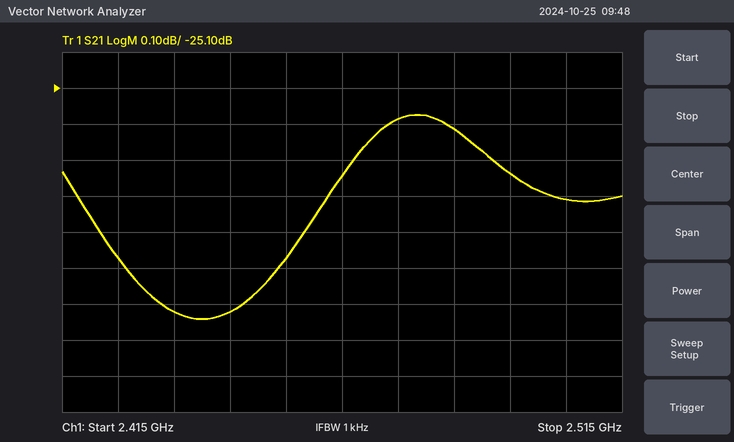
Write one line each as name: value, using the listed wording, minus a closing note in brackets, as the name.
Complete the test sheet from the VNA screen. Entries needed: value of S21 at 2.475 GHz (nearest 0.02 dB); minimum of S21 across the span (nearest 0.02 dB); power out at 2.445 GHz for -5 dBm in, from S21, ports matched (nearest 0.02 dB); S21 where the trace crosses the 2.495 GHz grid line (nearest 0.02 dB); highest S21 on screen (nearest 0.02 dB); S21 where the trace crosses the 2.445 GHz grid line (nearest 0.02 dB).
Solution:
value of S21 at 2.475 GHz: -25.18 dB
minimum of S21 across the span: -25.74 dB
power out at 2.445 GHz for -5 dBm in, from S21, ports matched: -30.72 dBm
S21 where the trace crosses the 2.495 GHz grid line: -25.34 dB
highest S21 on screen: -25.18 dB
S21 where the trace crosses the 2.445 GHz grid line: -25.72 dB
